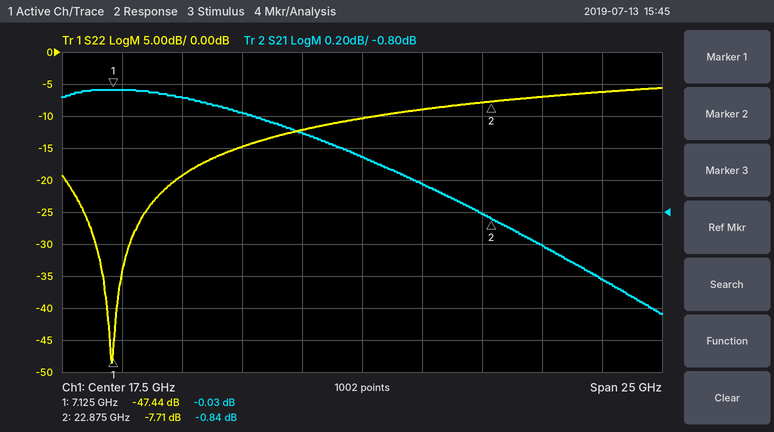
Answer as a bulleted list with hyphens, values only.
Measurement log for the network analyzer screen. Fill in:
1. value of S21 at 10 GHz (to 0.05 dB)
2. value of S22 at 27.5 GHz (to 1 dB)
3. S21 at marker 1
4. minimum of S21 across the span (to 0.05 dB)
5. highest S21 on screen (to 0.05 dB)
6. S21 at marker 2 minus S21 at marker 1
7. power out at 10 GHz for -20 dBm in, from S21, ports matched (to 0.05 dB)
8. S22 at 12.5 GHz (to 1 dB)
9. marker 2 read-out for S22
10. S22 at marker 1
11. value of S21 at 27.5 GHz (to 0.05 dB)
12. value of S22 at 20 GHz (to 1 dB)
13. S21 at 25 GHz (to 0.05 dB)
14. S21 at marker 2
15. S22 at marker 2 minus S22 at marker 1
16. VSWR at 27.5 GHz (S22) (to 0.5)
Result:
- -0.10 dB
- -6 dB
- -0.03 dB
- -1.45 dB
- -0.05 dB
- -0.81 dB
- -20.10 dBm
- -15 dB
- -7.71 dB
- -47.44 dB
- -1.20 dB
- -9 dB
- -1.00 dB
- -0.84 dB
- 39.73 dB
- 3.0
